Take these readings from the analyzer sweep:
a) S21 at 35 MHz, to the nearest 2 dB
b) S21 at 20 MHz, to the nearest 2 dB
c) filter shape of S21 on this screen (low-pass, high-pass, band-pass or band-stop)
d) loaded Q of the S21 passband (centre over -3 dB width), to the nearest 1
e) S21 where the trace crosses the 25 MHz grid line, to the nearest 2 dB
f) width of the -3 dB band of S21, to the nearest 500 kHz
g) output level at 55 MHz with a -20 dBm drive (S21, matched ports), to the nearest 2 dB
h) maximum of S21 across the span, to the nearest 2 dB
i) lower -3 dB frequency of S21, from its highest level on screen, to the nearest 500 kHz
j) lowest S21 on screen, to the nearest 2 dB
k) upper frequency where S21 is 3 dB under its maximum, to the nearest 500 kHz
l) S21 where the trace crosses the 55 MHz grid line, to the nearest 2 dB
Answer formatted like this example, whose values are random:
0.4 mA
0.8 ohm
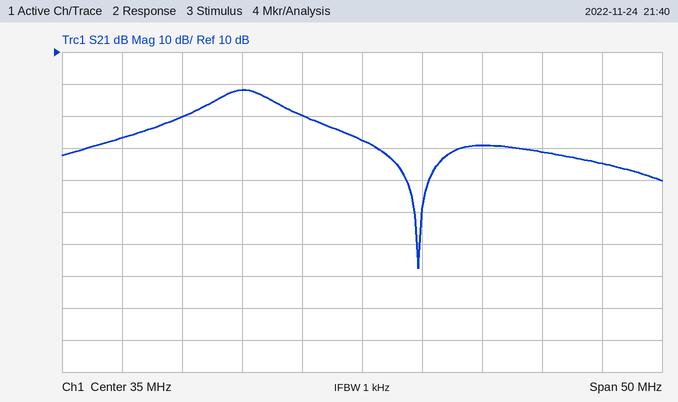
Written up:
-18 dB
-10 dB
band-pass
6
-2 dB
4.5 MHz
-44 dBm
-2 dB
23.0 MHz
-58 dB
27.5 MHz
-24 dB
